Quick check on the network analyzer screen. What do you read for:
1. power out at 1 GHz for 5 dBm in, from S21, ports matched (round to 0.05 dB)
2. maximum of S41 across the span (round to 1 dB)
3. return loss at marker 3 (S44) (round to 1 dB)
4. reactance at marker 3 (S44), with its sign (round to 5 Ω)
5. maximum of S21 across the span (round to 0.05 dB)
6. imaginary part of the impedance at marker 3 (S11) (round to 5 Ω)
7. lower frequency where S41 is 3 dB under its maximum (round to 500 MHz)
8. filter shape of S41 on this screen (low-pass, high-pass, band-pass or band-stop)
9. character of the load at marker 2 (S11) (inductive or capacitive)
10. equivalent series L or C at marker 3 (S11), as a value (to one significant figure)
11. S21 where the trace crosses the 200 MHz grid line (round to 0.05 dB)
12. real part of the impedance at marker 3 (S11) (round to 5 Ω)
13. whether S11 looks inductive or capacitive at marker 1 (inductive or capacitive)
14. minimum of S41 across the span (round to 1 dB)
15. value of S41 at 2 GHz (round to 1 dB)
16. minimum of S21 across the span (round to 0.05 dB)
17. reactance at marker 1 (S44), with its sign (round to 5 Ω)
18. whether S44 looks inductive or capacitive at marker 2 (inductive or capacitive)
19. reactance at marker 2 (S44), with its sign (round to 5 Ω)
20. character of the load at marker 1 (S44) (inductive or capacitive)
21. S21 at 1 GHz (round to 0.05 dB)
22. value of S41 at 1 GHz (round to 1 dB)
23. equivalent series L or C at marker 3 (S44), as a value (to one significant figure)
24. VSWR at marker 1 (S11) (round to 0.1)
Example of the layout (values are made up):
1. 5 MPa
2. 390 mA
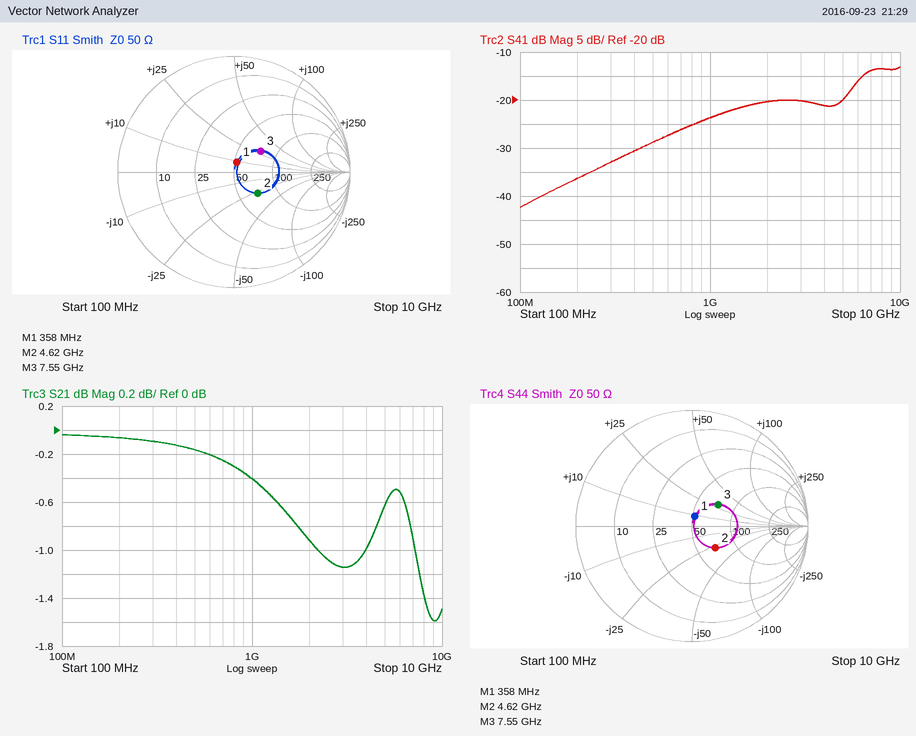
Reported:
1. 4.60 dBm
2. -13 dB
3. 11 dB
4. +30 Ω
5. -0.05 dB
6. +30 Ω
7. 6.0 GHz
8. high-pass
9. capacitive
10. 600 pH
11. -0.05 dB
12. 75 Ω
13. inductive
14. -42 dB
15. -20 dB
16. -1.60 dB
17. +10 Ω
18. capacitive
19. -30 Ω
20. inductive
21. -0.40 dB
22. -24 dB
23. 600 pH
24. 1.2
